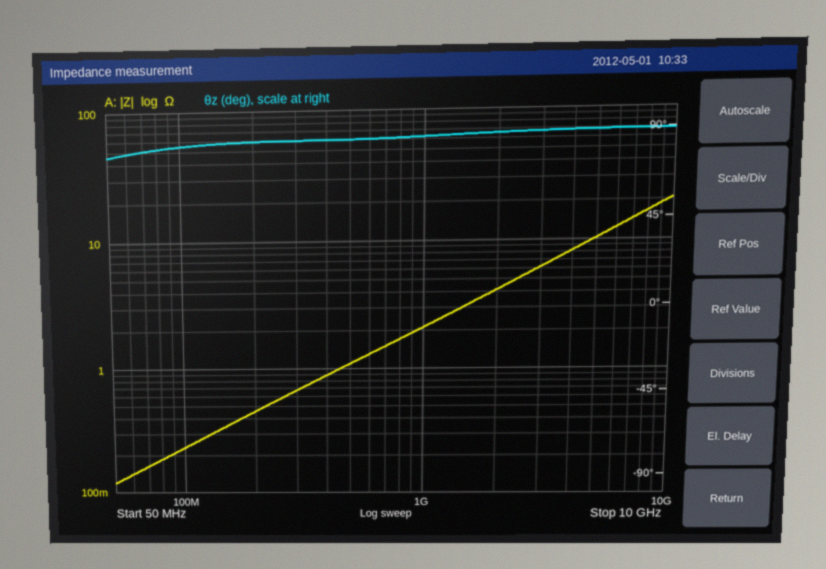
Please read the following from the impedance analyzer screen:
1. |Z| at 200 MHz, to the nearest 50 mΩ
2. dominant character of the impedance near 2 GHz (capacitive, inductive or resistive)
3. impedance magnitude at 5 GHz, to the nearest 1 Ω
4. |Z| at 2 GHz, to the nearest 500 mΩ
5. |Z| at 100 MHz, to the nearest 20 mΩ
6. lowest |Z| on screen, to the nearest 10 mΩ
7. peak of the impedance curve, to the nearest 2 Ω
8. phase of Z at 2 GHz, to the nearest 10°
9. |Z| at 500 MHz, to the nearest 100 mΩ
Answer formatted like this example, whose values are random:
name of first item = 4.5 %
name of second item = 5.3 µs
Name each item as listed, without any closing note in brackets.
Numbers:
|Z| at 200 MHz, to the nearest 50 mΩ = 450 mΩ
dominant character of the impedance near 2 GHz = inductive
impedance magnitude at 5 GHz, to the nearest 1 Ω = 10 Ω
|Z| at 2 GHz, to the nearest 500 mΩ = 4.0 Ω
|Z| at 100 MHz, to the nearest 20 mΩ = 240 mΩ
lowest |Z| on screen, to the nearest 10 mΩ = 120 mΩ
peak of the impedance curve, to the nearest 2 Ω = 20 Ω
phase of Z at 2 GHz, to the nearest 10° = 90°
|Z| at 500 MHz, to the nearest 100 mΩ = 1.1 Ω
